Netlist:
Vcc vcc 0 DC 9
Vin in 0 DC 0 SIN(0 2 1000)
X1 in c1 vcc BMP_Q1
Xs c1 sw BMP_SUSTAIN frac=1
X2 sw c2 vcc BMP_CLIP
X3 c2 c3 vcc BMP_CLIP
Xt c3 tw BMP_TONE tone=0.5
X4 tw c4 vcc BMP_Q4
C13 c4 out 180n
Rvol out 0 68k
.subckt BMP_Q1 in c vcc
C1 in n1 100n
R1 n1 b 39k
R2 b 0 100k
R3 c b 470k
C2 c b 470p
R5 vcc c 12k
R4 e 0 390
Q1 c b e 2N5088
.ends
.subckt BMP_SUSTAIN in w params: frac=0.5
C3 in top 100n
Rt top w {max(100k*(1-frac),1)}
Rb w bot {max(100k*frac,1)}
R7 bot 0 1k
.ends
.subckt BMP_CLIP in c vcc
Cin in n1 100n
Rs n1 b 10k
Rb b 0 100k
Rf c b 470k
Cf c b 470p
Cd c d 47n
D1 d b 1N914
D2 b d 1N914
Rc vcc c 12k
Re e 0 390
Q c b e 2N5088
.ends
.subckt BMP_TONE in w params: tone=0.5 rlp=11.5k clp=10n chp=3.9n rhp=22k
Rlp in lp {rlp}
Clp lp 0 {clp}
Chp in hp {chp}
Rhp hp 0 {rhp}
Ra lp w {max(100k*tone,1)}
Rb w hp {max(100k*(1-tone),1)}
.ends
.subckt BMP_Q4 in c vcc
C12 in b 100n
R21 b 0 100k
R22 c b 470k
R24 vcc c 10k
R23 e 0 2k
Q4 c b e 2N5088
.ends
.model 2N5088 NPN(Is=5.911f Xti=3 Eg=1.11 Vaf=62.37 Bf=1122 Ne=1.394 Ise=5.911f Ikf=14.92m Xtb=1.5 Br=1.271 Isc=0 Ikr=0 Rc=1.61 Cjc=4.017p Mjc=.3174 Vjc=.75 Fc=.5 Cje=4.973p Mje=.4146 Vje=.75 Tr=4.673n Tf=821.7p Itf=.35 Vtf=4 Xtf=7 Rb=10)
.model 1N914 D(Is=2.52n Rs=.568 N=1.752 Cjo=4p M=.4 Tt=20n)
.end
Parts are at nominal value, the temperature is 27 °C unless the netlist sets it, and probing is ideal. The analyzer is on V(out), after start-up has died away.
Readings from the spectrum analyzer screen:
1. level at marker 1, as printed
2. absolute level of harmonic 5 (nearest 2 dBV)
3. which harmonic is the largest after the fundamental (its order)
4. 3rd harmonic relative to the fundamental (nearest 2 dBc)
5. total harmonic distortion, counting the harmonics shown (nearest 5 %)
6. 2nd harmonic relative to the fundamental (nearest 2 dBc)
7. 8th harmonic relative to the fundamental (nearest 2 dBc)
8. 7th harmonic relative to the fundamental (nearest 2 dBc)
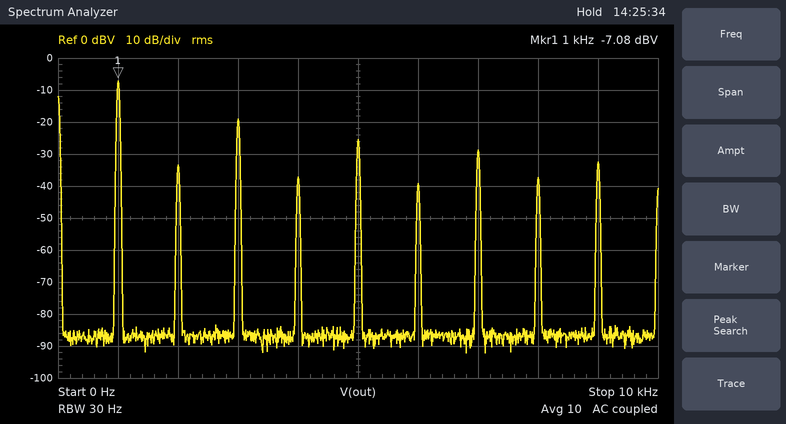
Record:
-7.08 dBV
-26 dBV
3
-12 dBc
30 %
-26 dBc
-30 dBc
-22 dBc
